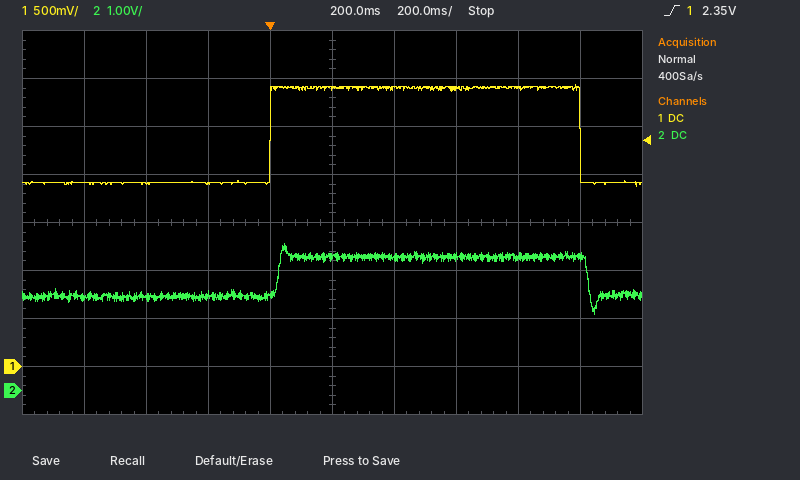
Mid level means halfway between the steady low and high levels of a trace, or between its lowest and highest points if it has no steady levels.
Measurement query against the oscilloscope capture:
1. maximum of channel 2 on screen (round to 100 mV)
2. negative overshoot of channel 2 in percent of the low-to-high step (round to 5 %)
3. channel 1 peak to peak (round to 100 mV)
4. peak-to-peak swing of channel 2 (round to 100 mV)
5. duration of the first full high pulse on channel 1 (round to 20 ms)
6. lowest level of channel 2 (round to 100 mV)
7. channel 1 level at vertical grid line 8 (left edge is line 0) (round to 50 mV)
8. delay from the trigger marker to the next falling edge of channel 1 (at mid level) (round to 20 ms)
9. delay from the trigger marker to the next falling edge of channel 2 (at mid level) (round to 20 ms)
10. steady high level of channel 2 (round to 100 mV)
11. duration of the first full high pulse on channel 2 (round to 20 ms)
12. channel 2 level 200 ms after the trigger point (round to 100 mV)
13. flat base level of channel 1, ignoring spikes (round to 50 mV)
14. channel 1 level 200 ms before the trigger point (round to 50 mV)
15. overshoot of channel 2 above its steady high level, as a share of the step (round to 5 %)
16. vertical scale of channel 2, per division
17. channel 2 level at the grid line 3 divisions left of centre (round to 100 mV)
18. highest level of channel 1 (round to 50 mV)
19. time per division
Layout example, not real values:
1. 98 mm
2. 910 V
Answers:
1. 3.1 V
2. 45 %
3. 1.10 V
4. 1.5 V
5. 1.00 s
6. 1.6 V
7. 2.90 V
8. 1.00 s
9. 1.02 s
10. 2.8 V
11. 1.00 s
12. 2.8 V
13. 1.90 V
14. 1.90 V
15. 35 %
16. 1 V
17. 1.9 V
18. 2.95 V
19. 200 ms
